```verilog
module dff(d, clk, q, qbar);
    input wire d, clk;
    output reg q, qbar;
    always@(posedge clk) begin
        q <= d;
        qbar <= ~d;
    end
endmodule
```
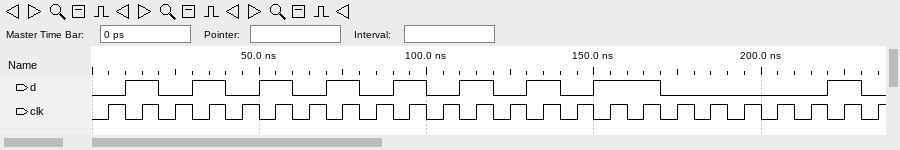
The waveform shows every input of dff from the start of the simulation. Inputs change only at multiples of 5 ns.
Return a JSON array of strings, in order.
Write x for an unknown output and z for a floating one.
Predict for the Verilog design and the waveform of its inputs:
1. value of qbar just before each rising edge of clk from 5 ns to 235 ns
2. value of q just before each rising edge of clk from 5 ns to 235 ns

["x 1 0 1 0 1 0 1 0 1 0 1 0 1 0 1 0 0 1 1 1 1 1 0", "x 0 1 0 1 0 1 0 1 0 1 0 1 0 1 0 1 1 0 0 0 0 0 1"]
